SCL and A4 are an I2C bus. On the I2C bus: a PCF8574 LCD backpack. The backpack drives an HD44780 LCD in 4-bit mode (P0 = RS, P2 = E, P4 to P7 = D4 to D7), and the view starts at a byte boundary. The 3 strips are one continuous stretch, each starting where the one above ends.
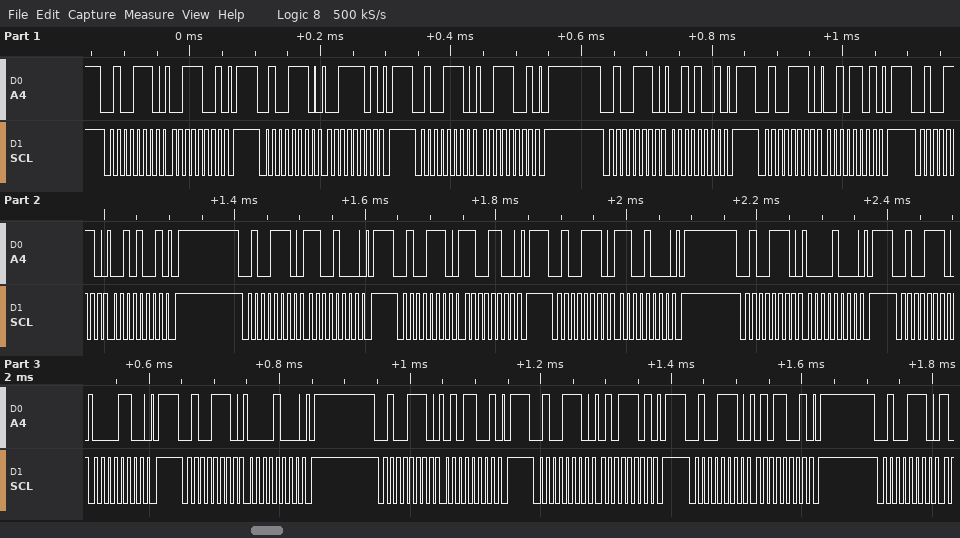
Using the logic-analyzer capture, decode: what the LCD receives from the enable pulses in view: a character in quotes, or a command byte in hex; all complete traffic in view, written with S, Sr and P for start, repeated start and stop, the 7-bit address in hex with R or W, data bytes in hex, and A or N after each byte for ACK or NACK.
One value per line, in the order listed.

'2' 0xC0
S 27W A 39 A P S 27W A 3D A P S 27W A 39 A P S 27W A 29 A P S 27W A 2D A P S 27W A 29 A P S 27W A C8 A P S 27W A CC A P S 27W A C8 A P S 27W A 08 A P S 27W A 0C A P S 27W A 08 A P S 27W A 59 A P S 27W A 5D A P S 27W A 59 A P S 27W A
